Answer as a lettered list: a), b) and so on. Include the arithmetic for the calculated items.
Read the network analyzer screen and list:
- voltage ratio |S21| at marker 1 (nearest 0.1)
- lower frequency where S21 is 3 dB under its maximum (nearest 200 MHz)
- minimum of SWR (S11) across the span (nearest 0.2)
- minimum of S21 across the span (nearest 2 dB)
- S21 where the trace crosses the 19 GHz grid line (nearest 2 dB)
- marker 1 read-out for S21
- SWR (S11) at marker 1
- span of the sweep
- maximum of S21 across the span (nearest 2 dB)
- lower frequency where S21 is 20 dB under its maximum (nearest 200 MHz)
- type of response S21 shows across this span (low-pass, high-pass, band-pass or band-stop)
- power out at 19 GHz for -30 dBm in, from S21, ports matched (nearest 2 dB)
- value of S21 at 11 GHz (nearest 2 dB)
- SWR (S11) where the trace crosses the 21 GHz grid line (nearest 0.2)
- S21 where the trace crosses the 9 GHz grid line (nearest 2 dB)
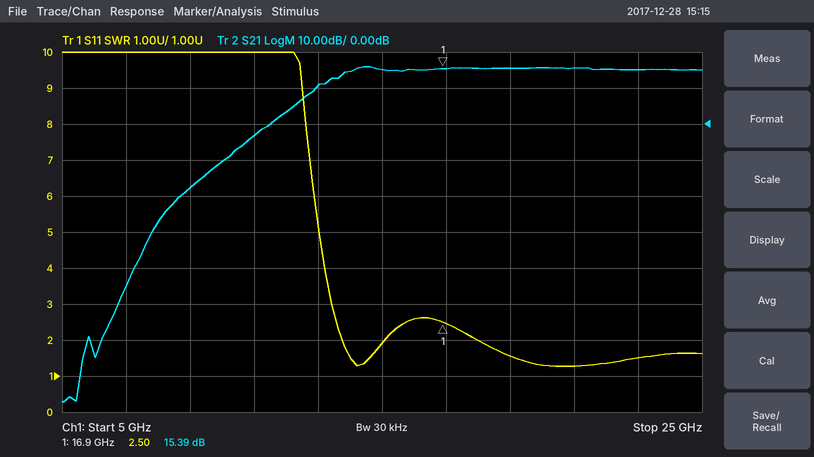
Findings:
a) 10^(15.39/20) ≈ 5.9
b) 13.6 GHz
c) 1.2
d) -78 dB
e) 16 dB
f) 15.39 dB
g) 2.50
h) 20 GHz
i) 16 dB
j) 10.8 GHz
k) high-pass
l) -30 dBm + (16 dB) = -14 dBm
m) -4 dB
n) 1.2
o) -18 dB
